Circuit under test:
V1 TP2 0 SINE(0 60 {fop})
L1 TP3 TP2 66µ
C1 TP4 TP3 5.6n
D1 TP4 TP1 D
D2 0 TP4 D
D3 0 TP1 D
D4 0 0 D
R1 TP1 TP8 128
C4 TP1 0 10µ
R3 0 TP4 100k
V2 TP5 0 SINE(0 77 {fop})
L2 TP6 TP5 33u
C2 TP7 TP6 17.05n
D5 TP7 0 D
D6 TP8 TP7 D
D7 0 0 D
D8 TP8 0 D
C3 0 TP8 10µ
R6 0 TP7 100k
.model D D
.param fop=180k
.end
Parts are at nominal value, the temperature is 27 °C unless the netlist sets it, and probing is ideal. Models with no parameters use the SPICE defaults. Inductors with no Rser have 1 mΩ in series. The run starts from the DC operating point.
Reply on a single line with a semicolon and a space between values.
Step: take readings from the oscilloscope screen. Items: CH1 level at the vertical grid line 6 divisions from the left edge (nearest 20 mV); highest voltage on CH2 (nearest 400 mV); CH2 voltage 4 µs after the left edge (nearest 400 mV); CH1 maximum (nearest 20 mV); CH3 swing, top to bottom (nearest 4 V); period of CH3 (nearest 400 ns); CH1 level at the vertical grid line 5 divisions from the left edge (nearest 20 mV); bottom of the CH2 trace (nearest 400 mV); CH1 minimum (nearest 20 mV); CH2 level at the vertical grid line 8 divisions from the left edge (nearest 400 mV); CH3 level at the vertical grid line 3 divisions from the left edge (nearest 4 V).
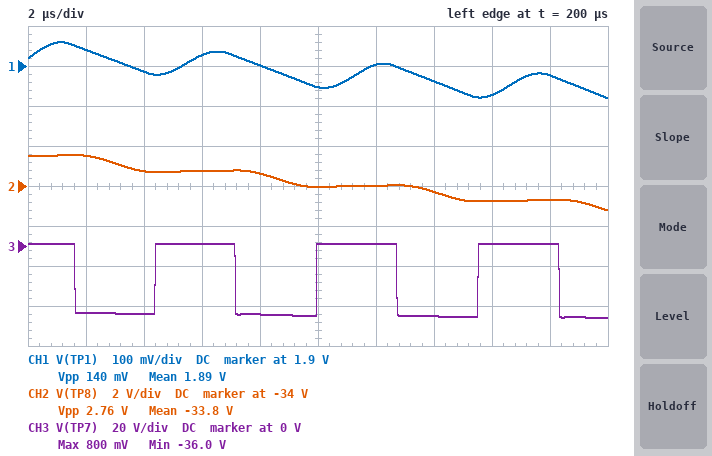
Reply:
1.90 V; -32.4 V; -33.2 V; 1.96 V; 36 V; 5.6 µs; 1.84 V; -35.2 V; 1.82 V; -34.8 V; 0 V
